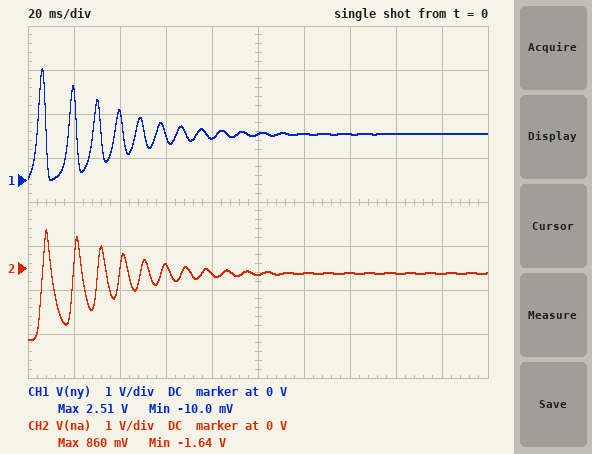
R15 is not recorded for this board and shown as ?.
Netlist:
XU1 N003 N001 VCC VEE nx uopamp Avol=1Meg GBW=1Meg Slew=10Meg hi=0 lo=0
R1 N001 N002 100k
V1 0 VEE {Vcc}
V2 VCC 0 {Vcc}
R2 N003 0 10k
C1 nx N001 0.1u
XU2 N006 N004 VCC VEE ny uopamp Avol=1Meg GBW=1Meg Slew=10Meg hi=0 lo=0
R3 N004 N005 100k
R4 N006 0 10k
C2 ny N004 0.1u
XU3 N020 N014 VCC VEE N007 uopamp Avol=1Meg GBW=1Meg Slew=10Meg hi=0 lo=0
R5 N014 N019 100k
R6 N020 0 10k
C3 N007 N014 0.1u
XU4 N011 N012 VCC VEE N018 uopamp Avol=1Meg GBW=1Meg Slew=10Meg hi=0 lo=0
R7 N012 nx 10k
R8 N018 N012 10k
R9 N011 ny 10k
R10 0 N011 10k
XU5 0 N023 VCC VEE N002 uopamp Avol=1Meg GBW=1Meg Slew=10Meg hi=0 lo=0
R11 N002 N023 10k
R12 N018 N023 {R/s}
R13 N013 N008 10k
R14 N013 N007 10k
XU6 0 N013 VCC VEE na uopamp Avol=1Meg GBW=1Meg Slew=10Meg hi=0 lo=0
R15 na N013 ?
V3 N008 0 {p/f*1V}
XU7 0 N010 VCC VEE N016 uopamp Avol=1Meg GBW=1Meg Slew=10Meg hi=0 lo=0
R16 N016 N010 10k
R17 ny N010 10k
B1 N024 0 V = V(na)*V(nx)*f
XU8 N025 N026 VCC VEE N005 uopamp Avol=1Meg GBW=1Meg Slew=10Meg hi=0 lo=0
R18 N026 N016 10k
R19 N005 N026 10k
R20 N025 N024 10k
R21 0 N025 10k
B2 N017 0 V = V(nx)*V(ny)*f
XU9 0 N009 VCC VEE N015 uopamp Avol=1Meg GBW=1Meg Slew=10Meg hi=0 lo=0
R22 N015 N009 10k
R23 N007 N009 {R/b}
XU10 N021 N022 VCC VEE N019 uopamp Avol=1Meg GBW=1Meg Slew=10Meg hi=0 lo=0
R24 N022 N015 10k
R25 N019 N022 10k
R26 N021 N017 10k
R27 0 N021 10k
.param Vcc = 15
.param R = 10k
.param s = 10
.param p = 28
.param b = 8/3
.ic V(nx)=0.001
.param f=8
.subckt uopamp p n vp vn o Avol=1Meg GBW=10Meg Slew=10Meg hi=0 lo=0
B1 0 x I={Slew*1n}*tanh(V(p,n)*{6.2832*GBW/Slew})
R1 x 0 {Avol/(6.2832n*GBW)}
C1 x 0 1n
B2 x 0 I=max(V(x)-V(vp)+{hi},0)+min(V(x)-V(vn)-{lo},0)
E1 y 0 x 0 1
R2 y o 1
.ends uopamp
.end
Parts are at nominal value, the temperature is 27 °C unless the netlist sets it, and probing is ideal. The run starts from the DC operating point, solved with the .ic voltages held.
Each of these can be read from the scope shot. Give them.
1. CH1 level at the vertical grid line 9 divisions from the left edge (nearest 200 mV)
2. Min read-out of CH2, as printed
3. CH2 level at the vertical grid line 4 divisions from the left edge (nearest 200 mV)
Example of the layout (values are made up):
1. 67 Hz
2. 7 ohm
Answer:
1. 1.0 V
2. -1.64 V
3. -200 mV
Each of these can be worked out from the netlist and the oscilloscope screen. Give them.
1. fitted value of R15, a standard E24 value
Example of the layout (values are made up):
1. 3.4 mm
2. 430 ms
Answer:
1. 4.7 kΩ
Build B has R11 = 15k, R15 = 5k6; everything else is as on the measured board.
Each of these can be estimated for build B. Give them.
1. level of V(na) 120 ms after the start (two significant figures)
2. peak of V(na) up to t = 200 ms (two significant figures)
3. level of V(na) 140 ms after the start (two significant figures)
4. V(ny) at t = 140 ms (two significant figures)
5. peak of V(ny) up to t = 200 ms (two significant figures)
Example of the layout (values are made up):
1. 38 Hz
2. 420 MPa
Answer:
1. -120 mV
2. 1.2 V
3. -130 mV
4. -1.0 V
5. 3.1 V
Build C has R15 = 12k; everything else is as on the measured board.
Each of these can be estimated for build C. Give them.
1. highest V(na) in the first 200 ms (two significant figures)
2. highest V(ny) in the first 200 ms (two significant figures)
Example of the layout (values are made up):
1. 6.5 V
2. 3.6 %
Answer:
1. 4.0 V
2. 4.4 V
